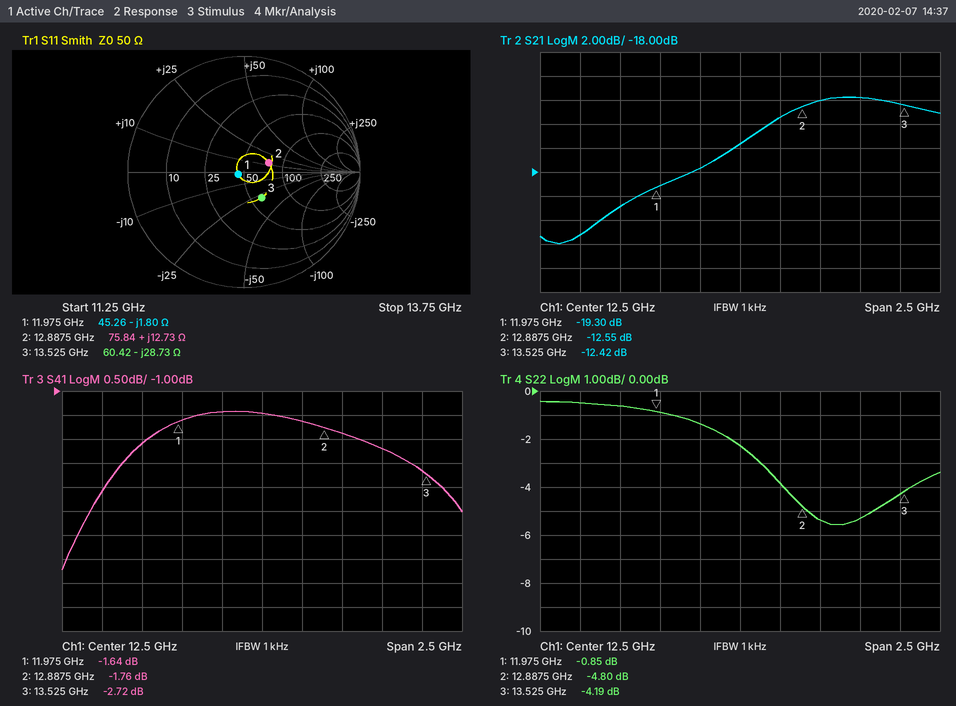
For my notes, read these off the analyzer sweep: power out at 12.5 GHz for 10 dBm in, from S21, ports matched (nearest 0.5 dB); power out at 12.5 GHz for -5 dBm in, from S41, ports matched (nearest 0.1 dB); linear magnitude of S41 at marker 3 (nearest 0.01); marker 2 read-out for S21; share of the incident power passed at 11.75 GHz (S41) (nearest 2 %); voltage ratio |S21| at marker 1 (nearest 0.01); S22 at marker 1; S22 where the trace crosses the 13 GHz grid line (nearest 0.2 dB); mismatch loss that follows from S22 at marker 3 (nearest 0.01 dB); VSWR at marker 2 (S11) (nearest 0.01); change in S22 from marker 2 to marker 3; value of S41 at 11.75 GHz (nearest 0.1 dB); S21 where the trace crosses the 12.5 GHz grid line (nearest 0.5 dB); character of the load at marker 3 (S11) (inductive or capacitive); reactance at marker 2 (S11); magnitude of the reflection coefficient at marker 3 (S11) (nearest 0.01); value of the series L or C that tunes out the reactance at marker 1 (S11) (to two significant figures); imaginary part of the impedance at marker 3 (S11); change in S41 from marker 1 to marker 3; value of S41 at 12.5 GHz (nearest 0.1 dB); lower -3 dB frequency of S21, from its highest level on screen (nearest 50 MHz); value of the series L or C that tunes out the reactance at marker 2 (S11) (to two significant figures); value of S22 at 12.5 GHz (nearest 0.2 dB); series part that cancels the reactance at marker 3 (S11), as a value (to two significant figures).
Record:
-5.5 dBm
-6.5 dBm
0.73
-12.55 dB
62 %
0.11
-0.85 dB
-5.4 dB
2.08 dB
1.59
0.61 dB
-2.1 dB
-15.5 dB
capacitive
+12.73 Ω
0.27
24 pH
-28.73 Ω
-1.08 dB
-1.5 dB
12.60 GHz
970 fF
-2.2 dB
340 pH
